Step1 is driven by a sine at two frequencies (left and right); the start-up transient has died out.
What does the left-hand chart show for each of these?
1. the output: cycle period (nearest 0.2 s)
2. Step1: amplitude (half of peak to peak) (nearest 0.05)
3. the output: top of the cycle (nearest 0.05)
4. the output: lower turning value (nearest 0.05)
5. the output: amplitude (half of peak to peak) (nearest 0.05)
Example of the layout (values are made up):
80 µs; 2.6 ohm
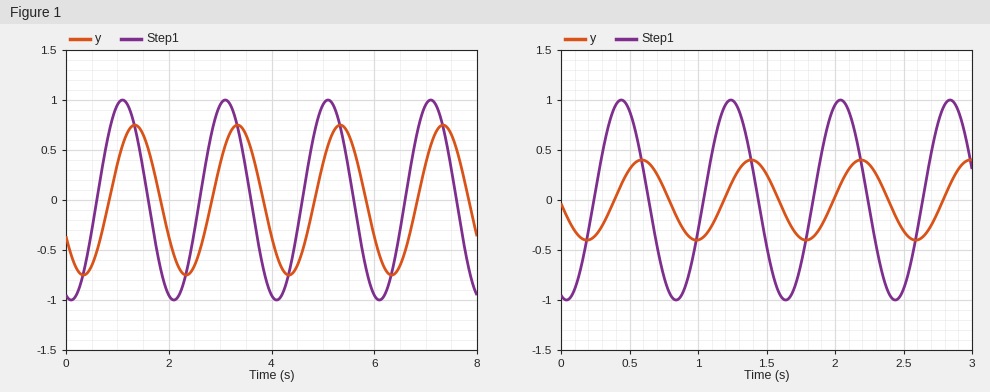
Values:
2.0 s; 1.00; 0.75; -0.75; 0.75
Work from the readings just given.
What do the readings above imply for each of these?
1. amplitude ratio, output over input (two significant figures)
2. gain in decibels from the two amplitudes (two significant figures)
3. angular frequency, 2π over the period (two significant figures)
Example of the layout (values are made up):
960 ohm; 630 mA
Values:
0.75; -2.5 dB; 3.1 rad/s
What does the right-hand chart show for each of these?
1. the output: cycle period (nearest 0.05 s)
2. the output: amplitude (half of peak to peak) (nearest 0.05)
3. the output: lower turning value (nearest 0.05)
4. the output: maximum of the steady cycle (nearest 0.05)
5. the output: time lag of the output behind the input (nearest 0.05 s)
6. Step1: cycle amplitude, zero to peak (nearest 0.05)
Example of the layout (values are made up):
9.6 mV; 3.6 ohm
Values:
0.80 s; 0.40; -0.40; 0.40; 0.15 s; 1.00
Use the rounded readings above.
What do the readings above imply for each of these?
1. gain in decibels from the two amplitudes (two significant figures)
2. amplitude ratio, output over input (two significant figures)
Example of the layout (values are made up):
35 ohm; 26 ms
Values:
-8.0 dB; 0.40
